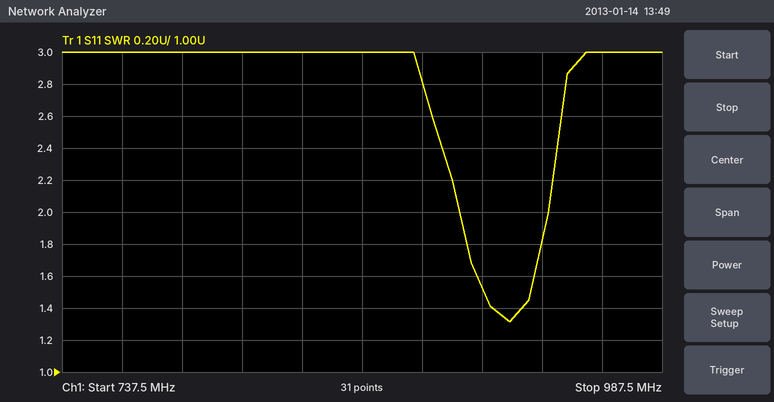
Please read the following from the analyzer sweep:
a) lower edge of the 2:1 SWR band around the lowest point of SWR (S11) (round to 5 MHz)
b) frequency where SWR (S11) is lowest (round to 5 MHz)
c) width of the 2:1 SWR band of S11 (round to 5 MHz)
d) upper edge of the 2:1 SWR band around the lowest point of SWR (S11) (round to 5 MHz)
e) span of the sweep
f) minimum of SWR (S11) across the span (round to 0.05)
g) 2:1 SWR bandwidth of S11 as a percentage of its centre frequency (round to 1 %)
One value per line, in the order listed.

905 MHz
925 MHz
35 MHz
940 MHz
250 MHz
1.30
4 %
